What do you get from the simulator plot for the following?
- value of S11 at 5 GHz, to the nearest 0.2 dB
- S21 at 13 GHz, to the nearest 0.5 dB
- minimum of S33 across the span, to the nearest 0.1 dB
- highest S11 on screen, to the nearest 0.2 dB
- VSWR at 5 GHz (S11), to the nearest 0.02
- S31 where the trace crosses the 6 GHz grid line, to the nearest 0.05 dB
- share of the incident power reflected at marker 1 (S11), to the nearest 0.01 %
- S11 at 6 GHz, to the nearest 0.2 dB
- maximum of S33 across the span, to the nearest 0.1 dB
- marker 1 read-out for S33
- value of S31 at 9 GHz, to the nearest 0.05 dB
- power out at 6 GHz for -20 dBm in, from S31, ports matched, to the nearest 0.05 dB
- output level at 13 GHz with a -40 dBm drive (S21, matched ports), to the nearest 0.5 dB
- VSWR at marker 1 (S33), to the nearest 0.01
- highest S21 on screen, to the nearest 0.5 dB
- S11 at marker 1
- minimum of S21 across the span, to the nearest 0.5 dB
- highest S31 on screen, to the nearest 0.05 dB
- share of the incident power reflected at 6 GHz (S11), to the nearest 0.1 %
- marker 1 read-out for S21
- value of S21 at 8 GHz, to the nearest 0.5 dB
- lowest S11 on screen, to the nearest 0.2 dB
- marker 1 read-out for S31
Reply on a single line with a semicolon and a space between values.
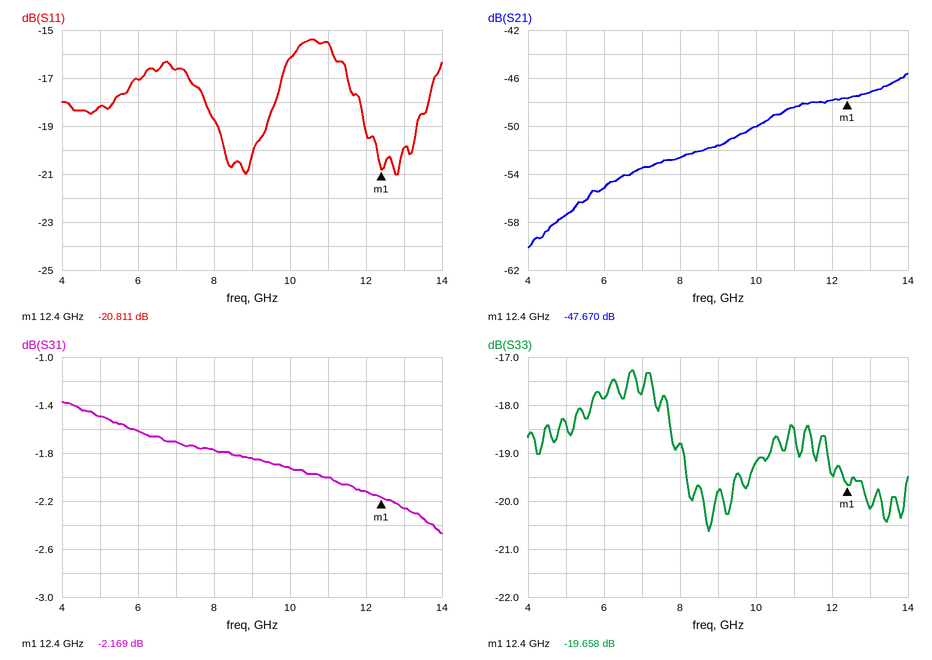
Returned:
-18.2 dB; -47.0 dB; -20.6 dB; -15.4 dB; 1.28; -1.60 dB; 0.83 %; -17.0 dB; -17.3 dB; -19.658 dB; -1.85 dB; -21.60 dBm; -87.0 dBm; 1.23; -45.5 dB; -20.811 dB; -60.0 dB; -1.35 dB; 2.0 %; -47.670 dB; -52.5 dB; -21.0 dB; -2.169 dB
